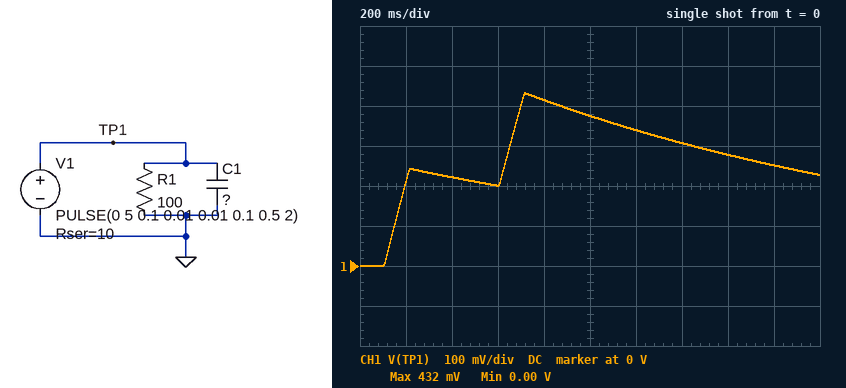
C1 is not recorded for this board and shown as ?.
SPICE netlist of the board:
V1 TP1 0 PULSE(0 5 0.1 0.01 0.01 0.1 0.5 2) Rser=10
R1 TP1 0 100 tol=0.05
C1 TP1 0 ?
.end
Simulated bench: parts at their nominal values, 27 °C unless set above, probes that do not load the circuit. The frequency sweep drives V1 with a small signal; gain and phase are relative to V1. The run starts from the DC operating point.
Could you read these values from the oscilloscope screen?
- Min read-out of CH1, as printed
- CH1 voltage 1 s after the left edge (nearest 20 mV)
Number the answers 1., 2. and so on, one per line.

1. 0.00 V
2. 380 mV
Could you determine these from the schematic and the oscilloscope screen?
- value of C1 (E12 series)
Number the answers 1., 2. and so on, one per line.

1. 220 mF
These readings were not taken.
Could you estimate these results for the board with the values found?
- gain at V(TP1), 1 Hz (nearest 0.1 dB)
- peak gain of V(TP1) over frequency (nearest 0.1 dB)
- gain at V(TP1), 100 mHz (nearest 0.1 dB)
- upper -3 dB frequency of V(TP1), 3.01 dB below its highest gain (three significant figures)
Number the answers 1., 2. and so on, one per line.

1. -22.8 dB
2. -0.8 dB
3. -4.9 dB
4. 79.6 mHz
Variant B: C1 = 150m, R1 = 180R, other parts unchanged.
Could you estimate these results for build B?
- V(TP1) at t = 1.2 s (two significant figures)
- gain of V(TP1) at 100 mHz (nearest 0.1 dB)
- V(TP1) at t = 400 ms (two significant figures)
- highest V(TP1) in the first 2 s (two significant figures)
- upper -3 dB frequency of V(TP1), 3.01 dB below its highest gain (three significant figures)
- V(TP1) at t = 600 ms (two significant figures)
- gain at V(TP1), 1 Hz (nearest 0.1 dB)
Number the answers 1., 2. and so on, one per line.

1. 430 mV
2. -3.0 dB
3. 310 mV
4. 600 mV
5. 112 mHz
6. 270 mV
7. -19.5 dB
